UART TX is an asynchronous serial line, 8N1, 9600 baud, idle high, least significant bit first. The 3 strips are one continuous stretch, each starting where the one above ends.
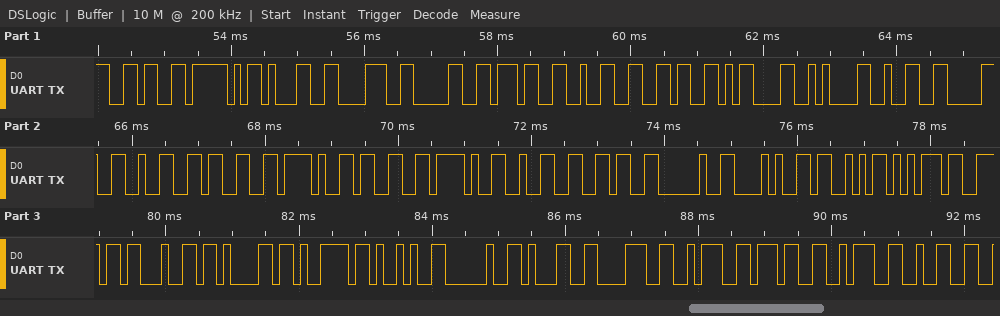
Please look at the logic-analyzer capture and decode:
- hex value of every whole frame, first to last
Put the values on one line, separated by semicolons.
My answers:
0x36 0x5F 0x31 0x38 0x30 0x37 0x32 0x36 0x0D 0x0A 0x32 0x30 0x32 0x33 0x2F 0x33 0x2F 0x32 0x36 0x20 0x28 0x53 0x75 0x6E 0x64 0x61 0x79 0x29 0x20 0x31 0x38 0x3A 0x37 0x3A 0x32
